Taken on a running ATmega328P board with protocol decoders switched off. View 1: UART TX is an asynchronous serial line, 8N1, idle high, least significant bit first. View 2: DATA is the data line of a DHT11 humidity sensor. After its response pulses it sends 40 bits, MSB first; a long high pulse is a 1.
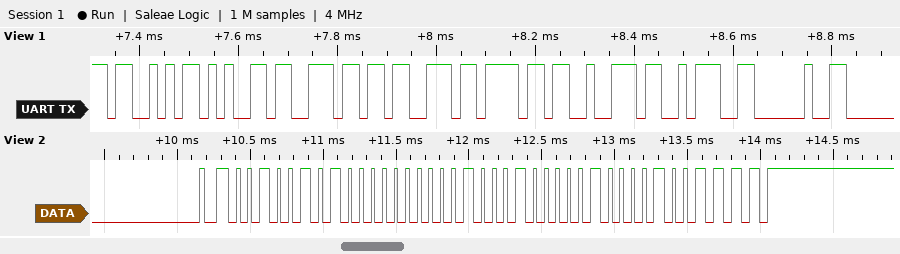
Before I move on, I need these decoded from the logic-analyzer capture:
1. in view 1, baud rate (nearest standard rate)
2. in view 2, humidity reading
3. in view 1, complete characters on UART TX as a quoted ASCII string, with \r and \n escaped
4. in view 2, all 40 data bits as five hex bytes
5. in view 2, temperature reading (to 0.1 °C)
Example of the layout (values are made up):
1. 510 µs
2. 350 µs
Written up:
1. 57600 baud
2. 37 %
3. "Sensor: "
4. 25 00 22 08 4F
5. 34.8 °C
